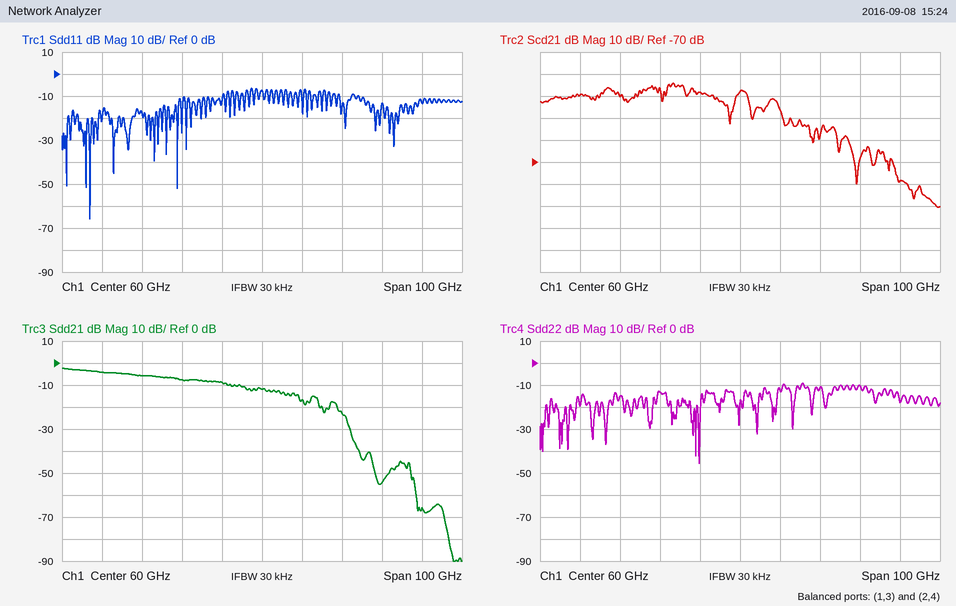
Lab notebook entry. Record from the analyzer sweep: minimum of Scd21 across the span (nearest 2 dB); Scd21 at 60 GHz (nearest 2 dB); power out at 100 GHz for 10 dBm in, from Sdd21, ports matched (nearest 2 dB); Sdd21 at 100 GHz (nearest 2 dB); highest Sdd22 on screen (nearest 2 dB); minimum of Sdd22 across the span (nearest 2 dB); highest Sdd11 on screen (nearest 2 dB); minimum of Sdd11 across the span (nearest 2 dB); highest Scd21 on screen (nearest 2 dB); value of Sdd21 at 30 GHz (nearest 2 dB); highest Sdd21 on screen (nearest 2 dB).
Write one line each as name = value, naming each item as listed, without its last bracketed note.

minimum of Scd21 across the span = -90 dB
Scd21 at 60 GHz = -38 dB
power out at 100 GHz for 10 dBm in, from Sdd21, ports matched = -56 dBm
Sdd21 at 100 GHz = -66 dB
highest Sdd22 on screen = -10 dB
minimum of Sdd22 across the span = -46 dB
highest Sdd11 on screen = -6 dB
minimum of Sdd11 across the span = -66 dB
highest Scd21 on screen = -34 dB
value of Sdd21 at 30 GHz = -6 dB
highest Sdd21 on screen = -2 dB
